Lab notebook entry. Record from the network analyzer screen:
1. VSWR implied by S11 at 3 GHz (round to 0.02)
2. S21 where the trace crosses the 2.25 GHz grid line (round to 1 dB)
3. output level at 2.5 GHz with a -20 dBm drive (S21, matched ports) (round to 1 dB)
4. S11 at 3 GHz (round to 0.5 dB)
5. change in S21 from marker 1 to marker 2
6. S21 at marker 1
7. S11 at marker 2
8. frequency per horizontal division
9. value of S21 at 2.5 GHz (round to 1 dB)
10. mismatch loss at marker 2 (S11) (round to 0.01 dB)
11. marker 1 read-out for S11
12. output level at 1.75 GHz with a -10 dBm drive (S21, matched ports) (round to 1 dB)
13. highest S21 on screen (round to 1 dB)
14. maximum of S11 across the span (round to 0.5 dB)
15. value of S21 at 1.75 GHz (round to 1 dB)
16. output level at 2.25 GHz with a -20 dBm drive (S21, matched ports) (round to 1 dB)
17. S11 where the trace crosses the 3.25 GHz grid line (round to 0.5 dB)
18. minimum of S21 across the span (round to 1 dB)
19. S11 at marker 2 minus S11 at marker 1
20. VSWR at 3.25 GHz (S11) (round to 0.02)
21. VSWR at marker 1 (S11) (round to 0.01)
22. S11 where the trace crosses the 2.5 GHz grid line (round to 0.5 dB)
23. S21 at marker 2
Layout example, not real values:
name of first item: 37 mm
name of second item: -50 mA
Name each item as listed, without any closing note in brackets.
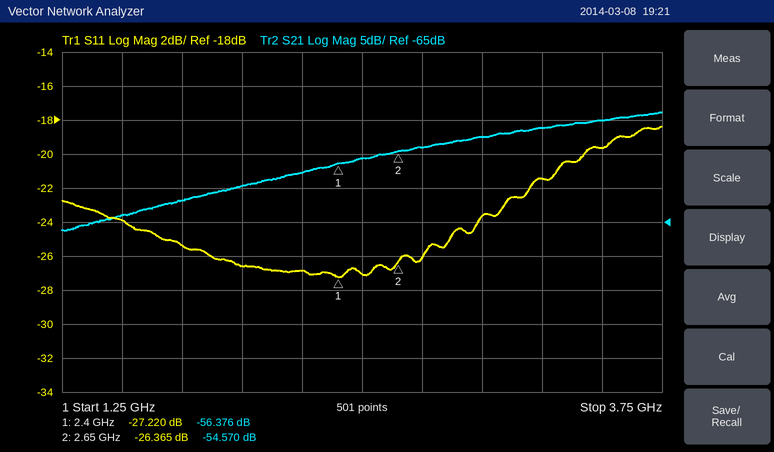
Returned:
VSWR implied by S11 at 3 GHz: 1.14
S21 where the trace crosses the 2.25 GHz grid line: -58 dB
output level at 2.5 GHz with a -20 dBm drive (S21, matched ports): -76 dBm
S11 at 3 GHz: -23.5 dB
change in S21 from marker 1 to marker 2: 1.806 dB
S21 at marker 1: -56.376 dB
S11 at marker 2: -26.365 dB
frequency per horizontal division: 250 MHz
value of S21 at 2.5 GHz: -56 dB
mismatch loss at marker 2 (S11): 0.01 dB
marker 1 read-out for S11: -27.220 dB
output level at 1.75 GHz with a -10 dBm drive (S21, matched ports): -72 dBm
highest S21 on screen: -49 dB
maximum of S11 across the span: -18.5 dB
value of S21 at 1.75 GHz: -62 dB
output level at 2.25 GHz with a -20 dBm drive (S21, matched ports): -78 dBm
S11 where the trace crosses the 3.25 GHz grid line: -21.5 dB
minimum of S21 across the span: -66 dB
S11 at marker 2 minus S11 at marker 1: 0.855 dB
VSWR at 3.25 GHz (S11): 1.18
VSWR at marker 1 (S11): 1.09
S11 where the trace crosses the 2.5 GHz grid line: -27.0 dB
S21 at marker 2: -54.570 dB
